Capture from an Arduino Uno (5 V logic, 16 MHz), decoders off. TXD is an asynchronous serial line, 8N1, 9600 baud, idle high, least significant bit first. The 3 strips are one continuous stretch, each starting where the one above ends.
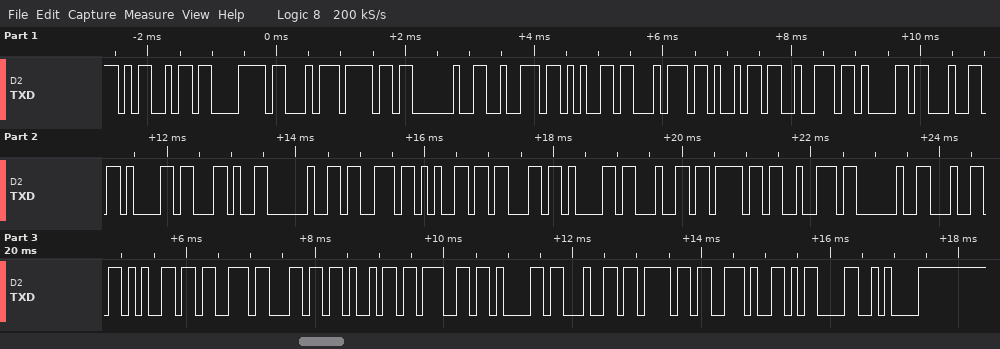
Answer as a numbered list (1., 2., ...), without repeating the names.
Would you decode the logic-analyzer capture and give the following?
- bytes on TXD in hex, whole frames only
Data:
1. 0x4D 0xC3 0xA3 0x6F 0x20 0x72 0x65 0x74 0x69 0x72 0x61 0x64 0x61 0x2C 0x20 0x73 0x65 0x63 0x61 0x64 0x6F 0x72 0x20 0x64 0x65 0x73 0x6C 0x69 0x67 0x61 0x64 0x6F 0x2E 0x0D 0x0A
